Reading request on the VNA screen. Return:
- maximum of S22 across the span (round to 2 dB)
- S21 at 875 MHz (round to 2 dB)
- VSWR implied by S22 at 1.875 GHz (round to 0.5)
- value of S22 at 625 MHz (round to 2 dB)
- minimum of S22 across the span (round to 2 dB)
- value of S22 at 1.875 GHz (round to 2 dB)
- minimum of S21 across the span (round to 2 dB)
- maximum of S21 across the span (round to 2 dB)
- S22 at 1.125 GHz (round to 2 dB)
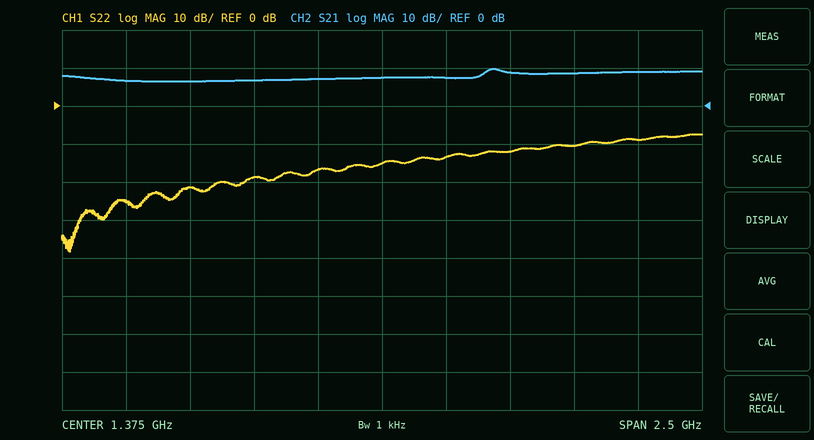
-8 dB
6 dB
1.5
-22 dB
-38 dB
-12 dB
6 dB
10 dB
-16 dB
